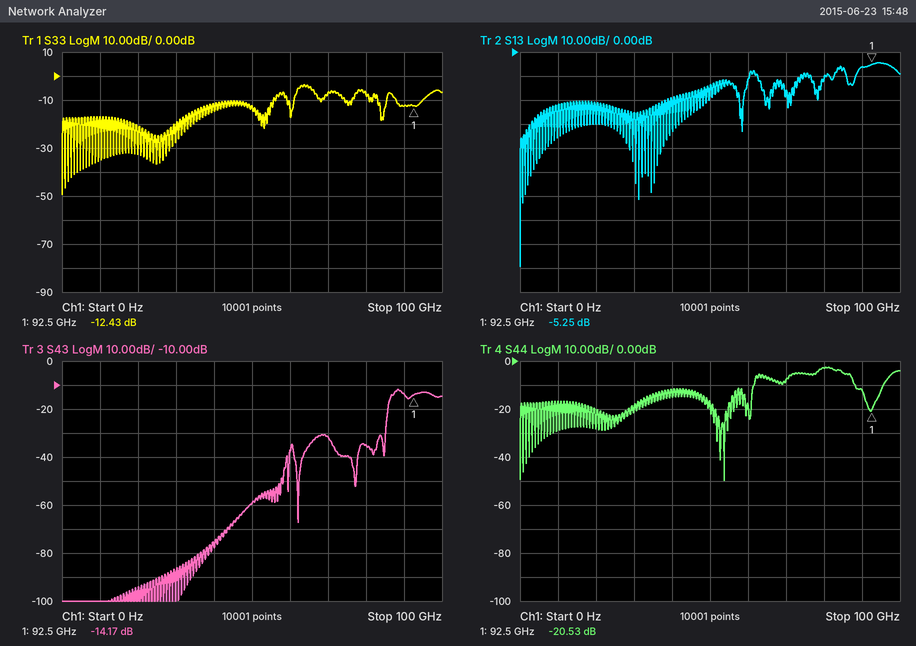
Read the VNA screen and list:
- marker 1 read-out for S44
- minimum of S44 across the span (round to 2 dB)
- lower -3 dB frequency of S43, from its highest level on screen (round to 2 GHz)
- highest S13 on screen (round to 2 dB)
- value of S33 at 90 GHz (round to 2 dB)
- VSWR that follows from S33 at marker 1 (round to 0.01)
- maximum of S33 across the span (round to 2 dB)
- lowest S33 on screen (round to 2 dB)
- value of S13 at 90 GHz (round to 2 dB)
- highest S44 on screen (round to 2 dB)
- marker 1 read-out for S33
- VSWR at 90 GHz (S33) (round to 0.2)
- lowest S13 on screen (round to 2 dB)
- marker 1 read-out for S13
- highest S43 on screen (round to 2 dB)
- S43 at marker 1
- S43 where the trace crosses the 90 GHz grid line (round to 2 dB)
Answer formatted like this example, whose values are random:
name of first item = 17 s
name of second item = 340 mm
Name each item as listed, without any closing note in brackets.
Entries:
marker 1 read-out for S44 = -20.53 dB
minimum of S44 across the span = -50 dB
lower -3 dB frequency of S43, from its highest level on screen = 86 GHz
highest S13 on screen = -4 dB
value of S33 at 90 GHz = -12 dB
VSWR that follows from S33 at marker 1 = 1.63
maximum of S33 across the span = -4 dB
lowest S33 on screen = -50 dB
value of S13 at 90 GHz = -6 dB
highest S44 on screen = -2 dB
marker 1 read-out for S33 = -12.43 dB
VSWR at 90 GHz (S33) = 1.6
lowest S13 on screen = -90 dB
marker 1 read-out for S13 = -5.25 dB
highest S43 on screen = -12 dB
S43 at marker 1 = -14.17 dB
S43 where the trace crosses the 90 GHz grid line = -14 dB
